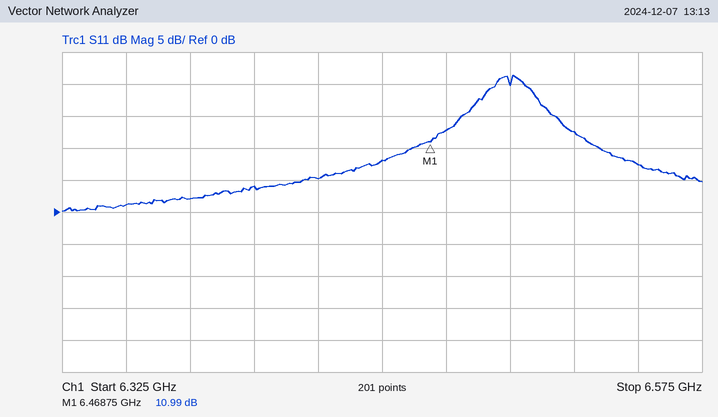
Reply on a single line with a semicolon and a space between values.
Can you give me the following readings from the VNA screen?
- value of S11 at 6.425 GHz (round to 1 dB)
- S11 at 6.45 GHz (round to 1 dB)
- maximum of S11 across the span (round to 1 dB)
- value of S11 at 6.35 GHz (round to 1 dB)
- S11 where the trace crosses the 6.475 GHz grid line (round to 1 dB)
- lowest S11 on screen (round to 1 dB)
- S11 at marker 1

5 dB; 8 dB; 21 dB; 1 dB; 13 dB; 0 dB; 10.99 dB
